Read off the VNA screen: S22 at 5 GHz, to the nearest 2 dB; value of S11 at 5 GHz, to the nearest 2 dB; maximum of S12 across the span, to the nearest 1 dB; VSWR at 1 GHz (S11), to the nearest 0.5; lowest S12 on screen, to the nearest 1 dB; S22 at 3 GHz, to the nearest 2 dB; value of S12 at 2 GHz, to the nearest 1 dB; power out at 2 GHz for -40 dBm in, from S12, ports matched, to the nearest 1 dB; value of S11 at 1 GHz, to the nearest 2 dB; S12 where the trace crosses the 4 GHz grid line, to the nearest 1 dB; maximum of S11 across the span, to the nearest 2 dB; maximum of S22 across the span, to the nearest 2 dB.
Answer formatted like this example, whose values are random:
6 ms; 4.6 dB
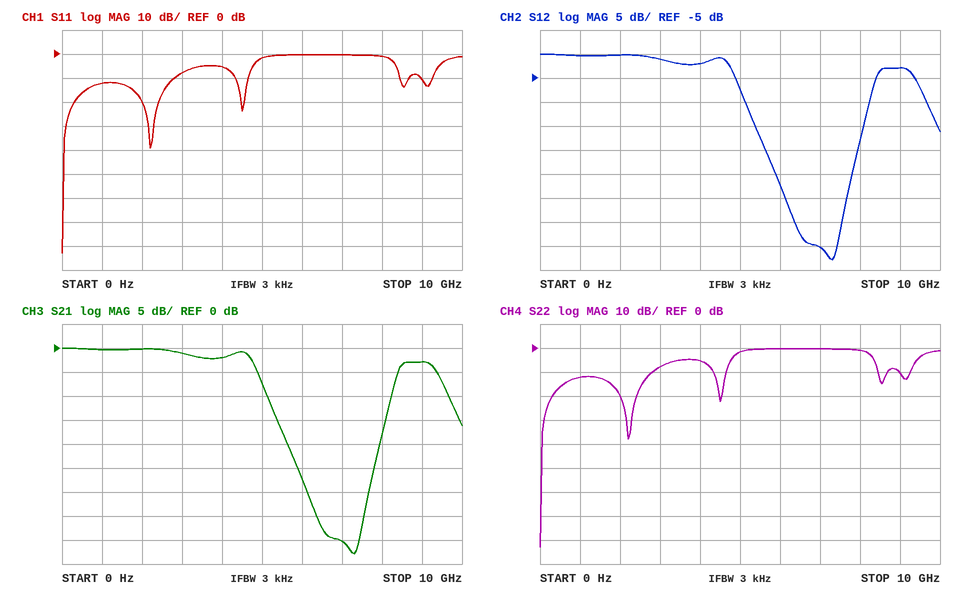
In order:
-2 dB; -2 dB; 0 dB; 1.5; -43 dB; -8 dB; 0 dB; -40 dBm; -12 dB; -2 dB; 0 dB; 0 dB
